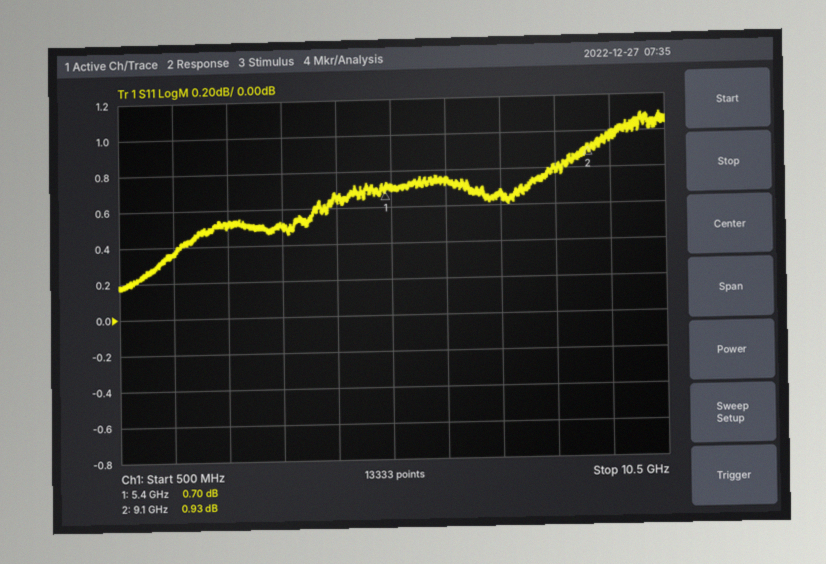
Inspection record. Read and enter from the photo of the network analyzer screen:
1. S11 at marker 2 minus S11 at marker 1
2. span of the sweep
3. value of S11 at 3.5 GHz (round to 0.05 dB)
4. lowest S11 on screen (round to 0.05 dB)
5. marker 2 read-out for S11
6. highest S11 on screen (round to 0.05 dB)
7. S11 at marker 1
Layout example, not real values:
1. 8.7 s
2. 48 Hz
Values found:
1. 0.23 dB
2. 10 GHz
3. 0.50 dB
4. 0.15 dB
5. 0.93 dB
6. 1.10 dB
7. 0.70 dB
